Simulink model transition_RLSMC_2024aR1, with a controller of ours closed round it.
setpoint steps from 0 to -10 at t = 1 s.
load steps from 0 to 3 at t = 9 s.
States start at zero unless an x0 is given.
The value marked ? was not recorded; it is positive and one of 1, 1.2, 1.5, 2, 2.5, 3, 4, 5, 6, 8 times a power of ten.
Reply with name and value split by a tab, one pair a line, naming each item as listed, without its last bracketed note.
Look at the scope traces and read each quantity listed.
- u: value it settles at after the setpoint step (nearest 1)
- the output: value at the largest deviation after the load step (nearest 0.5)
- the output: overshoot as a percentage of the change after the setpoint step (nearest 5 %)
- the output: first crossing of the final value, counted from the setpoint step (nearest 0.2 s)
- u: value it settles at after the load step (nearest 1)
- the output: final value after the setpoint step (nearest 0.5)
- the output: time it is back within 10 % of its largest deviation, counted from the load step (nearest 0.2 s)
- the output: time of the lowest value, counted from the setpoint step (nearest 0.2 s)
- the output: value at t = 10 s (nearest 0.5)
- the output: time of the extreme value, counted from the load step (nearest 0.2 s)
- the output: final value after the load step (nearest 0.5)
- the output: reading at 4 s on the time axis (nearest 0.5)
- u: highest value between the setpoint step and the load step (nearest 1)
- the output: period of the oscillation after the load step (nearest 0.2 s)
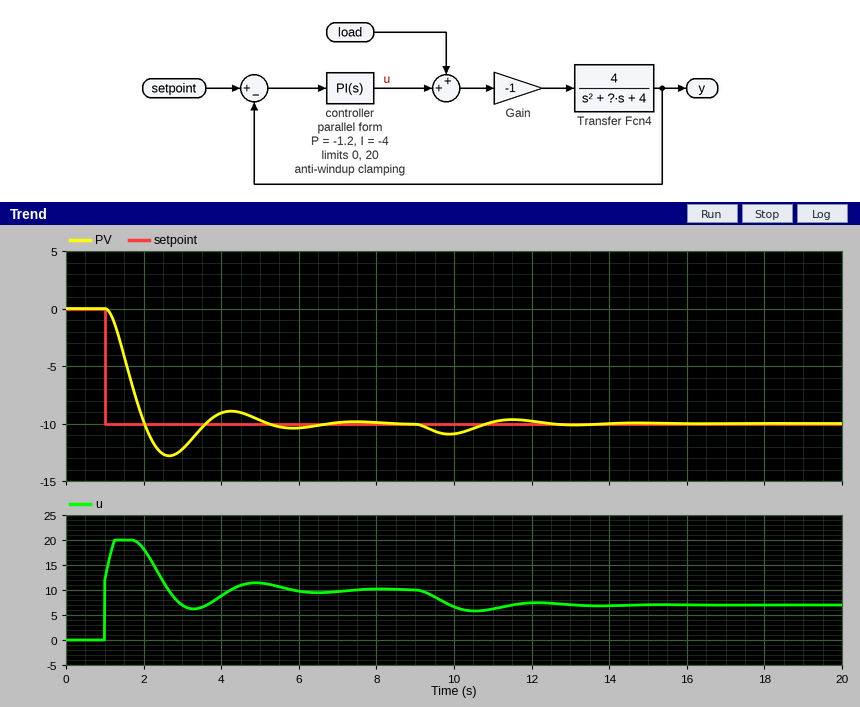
u: value it settles at after the setpoint step	10
the output: value at the largest deviation after the load step	-11.0
the output: overshoot as a percentage of the change after the setpoint step	30 %
the output: first crossing of the final value, counted from the setpoint step	1.0 s
u: value it settles at after the load step	7
the output: final value after the setpoint step	-10.0
the output: time it is back within 10 % of its largest deviation, counted from the load step	4.6 s
the output: time of the lowest value, counted from the setpoint step	1.6 s
the output: value at t = 10 s	-11.0
the output: time of the extreme value, counted from the load step	0.8 s
the output: final value after the load step	-10.0
the output: reading at 4 s on the time axis	-9.0
u: highest value between the setpoint step and the load step	20
the output: period of the oscillation after the load step	3.2 s
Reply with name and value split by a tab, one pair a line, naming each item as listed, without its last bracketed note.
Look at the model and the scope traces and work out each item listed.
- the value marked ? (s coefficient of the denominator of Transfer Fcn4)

the value marked ?	5
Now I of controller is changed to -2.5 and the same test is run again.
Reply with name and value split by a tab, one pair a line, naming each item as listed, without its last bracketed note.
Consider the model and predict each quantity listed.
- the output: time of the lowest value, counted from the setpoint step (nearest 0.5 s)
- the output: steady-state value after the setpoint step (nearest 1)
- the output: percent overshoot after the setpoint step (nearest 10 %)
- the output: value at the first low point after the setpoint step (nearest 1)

the output: time of the lowest value, counted from the setpoint step	2.0 s
the output: steady-state value after the setpoint step	-10
the output: percent overshoot after the setpoint step	20 %
the output: value at the first low point after the setpoint step	-12
